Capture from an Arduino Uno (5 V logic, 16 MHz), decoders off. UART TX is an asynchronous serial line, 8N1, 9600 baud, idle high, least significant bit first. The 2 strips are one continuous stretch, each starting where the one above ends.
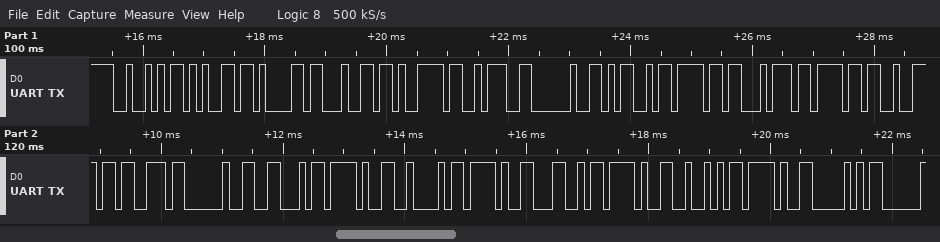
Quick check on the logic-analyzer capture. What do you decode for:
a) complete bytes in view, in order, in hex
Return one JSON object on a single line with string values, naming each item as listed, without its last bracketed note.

{"complete bytes in view, in order, in hex": "0x52 0x65 0x61 0x64 0x79 0x3A 0x20 0x4D 0x6F 0x74 0x6F 0x72 0x73 0x20 0x46 0x2F 0x42 0x2F 0x4C 0x2F 0x52 0x2F 0x50"}
